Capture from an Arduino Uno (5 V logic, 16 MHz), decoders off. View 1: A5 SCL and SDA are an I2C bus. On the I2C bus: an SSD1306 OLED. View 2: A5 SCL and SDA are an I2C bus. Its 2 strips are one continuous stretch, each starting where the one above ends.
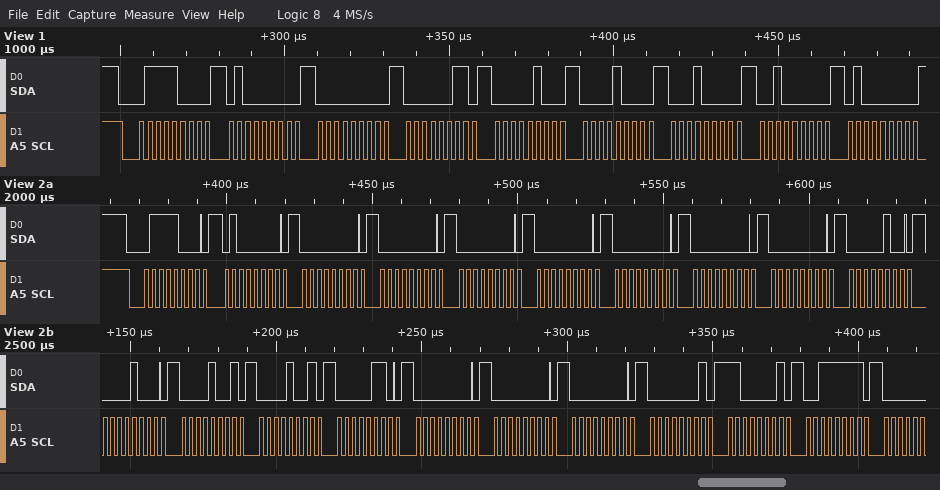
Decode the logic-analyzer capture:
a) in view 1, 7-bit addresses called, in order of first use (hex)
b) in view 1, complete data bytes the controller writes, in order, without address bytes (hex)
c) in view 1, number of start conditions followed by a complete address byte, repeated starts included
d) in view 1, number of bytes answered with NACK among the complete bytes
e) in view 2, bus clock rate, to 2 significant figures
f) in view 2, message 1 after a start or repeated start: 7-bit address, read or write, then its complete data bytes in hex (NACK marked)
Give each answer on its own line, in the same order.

0x3C
40 00 03 04 08 10 20 40
1
0
400 kHz
0x3C write: 40 00 00 00 00 00 00 00 04 08 09 09 06 00 00 00 01 C1 3F
